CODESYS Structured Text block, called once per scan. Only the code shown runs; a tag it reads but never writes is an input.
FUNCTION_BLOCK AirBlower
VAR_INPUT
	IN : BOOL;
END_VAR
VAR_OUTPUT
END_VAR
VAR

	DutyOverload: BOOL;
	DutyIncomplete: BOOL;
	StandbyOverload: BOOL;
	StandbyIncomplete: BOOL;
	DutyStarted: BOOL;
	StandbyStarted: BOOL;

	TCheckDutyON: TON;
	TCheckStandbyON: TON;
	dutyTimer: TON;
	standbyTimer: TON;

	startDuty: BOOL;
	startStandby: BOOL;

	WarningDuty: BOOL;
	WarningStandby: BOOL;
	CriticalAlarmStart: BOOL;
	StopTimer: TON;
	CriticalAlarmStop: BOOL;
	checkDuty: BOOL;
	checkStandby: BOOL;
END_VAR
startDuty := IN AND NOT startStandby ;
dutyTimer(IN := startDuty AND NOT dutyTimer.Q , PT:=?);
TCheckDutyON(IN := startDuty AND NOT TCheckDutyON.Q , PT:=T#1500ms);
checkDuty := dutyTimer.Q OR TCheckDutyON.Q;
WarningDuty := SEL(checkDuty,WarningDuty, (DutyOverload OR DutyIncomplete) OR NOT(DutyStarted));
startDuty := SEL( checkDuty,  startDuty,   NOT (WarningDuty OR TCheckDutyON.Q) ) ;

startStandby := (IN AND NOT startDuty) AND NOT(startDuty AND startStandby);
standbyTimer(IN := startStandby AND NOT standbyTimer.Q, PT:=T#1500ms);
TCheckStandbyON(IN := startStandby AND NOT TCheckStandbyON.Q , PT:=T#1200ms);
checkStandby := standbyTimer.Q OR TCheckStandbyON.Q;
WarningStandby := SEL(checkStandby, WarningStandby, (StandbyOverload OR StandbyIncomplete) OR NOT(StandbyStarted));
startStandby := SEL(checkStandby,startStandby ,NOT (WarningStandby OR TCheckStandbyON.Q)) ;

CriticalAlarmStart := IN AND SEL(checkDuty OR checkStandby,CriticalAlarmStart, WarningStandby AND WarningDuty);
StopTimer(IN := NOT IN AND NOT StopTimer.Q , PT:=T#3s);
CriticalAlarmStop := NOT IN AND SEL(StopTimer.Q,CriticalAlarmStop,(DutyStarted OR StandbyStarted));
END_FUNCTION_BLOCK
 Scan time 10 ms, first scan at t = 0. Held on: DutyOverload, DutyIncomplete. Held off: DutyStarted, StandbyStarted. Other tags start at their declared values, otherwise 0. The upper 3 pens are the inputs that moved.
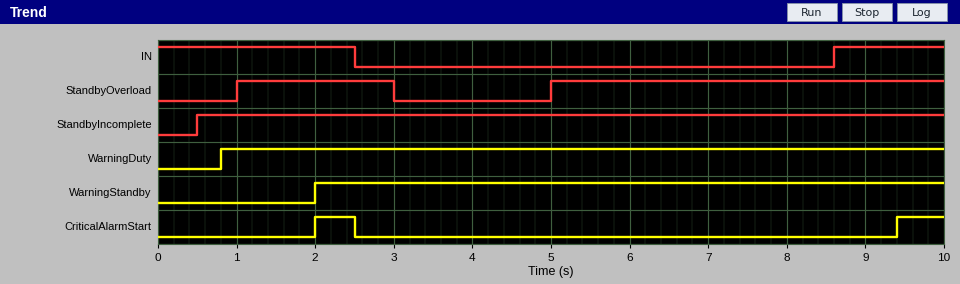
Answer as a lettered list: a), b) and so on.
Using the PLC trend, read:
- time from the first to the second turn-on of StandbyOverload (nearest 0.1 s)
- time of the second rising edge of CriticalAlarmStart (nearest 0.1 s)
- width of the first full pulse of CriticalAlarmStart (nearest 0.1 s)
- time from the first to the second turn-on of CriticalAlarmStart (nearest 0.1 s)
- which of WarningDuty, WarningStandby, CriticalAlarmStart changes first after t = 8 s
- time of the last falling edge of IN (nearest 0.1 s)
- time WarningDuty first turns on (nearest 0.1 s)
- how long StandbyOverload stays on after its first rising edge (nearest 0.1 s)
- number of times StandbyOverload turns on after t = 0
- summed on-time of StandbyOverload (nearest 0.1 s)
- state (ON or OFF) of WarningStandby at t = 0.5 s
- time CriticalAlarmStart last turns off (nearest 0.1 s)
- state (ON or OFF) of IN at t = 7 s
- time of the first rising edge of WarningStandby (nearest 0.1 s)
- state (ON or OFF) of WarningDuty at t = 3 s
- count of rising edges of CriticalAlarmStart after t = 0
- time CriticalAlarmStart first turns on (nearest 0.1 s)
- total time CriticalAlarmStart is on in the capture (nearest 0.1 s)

a) 4.0 s
b) 9.4 s
c) 0.5 s
d) 7.4 s
e) CriticalAlarmStart
f) 2.5 s
g) 0.8 s
h) 2.0 s
i) 2
j) 7.0 s
k) OFF
l) 2.5 s
m) OFF
n) 2.0 s
o) ON
p) 2
q) 2.0 s
r) 1.1 s
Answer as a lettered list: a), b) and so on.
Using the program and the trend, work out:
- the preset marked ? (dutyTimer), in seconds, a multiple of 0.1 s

a) 0.8 s
